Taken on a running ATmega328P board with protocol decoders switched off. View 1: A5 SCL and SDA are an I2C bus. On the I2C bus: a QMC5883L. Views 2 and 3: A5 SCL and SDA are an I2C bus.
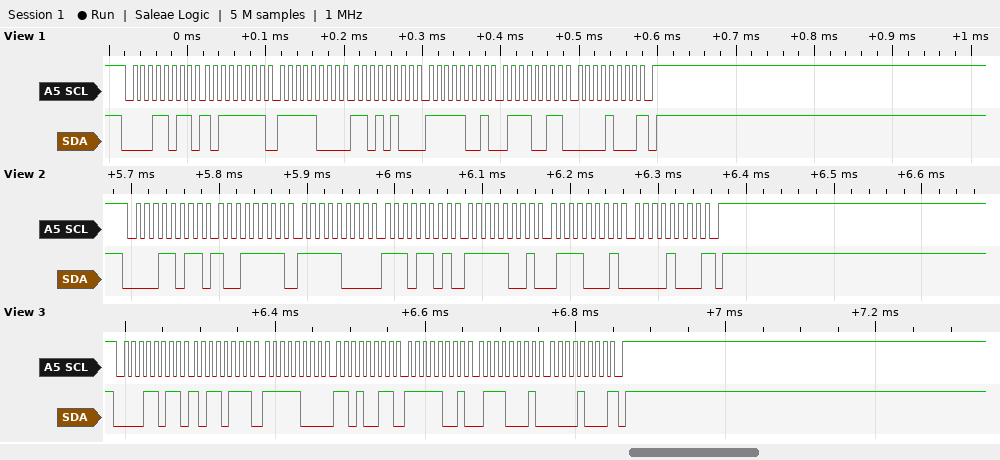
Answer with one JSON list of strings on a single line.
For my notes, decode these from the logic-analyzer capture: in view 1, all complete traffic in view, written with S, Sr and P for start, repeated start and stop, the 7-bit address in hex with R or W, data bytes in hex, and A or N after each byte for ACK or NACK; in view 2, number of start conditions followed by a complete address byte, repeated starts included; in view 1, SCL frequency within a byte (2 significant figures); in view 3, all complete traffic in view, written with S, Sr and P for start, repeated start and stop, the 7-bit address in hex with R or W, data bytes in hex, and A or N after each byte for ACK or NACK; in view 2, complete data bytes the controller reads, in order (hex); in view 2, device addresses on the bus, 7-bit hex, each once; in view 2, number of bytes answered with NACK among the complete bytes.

["S 0DR A BF A F8 A D4 A F9 A 73 A 08 N P", "1", "100 kHz", "S 0DR A B7 A F8 A D3 A F9 A 71 A 08 N P", "9F F8 ED F9 71 08", "0x0D", "1"]
